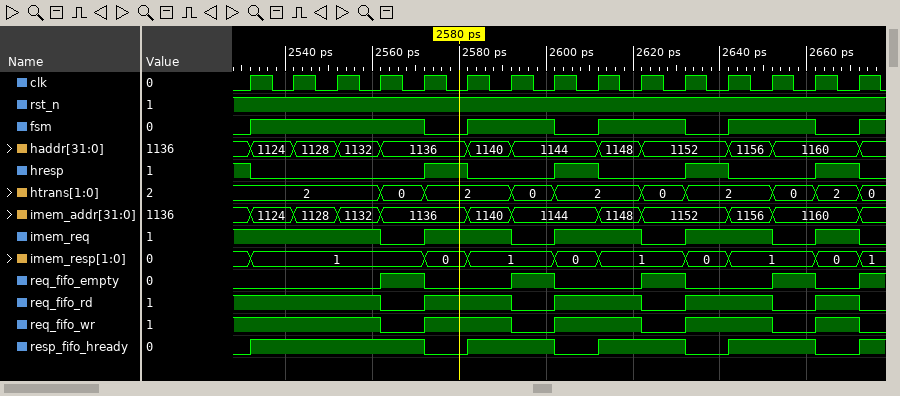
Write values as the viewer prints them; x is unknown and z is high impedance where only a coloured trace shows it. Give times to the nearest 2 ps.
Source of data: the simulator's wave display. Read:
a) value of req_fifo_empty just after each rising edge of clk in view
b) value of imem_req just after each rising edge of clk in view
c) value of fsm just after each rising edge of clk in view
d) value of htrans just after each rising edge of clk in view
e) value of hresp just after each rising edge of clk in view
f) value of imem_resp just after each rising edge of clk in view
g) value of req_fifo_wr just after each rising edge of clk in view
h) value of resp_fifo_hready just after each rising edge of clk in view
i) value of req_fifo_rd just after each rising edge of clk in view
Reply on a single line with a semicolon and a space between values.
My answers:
0 0 0 1 0 0 1 0 0 1 0 0 1 0 1; 1 1 1 0 1 1 0 1 1 0 1 1 0 1 0; 1 1 1 1 0 1 1 0 1 1 0 1 1 0 1; 2, 2, 2, 0, 2, 2, 0, 2, 2, 0, 2, 2, 0, 2, 0; 0 0 0 0 1 0 0 1 0 0 1 0 0 1 0; 1, 1, 1, 1, 0, 1, 1, 0, 1, 1, 0, 1, 1, 0, 1; 1 1 1 0 1 1 0 1 1 0 1 1 0 1 0; 1 1 1 1 0 1 1 0 1 1 0 1 1 0 1; 1 1 1 0 1 1 0 1 1 0 1 1 0 1 0
